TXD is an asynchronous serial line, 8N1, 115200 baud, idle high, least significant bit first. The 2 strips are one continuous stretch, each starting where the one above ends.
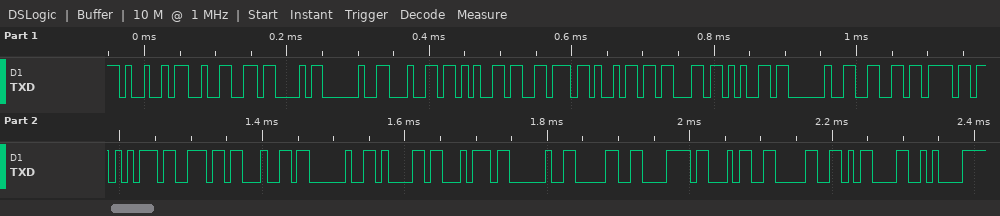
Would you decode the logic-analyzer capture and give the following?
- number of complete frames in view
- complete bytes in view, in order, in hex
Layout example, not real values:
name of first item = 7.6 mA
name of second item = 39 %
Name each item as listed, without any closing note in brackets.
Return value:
number of complete frames in view = 26
complete bytes in view, in order, in hex = 49 32 43 20 64 65 76 69 63 65 20 66 6F 75 6E 64 20 61 74 20 30 78 34 30 0D 0A
